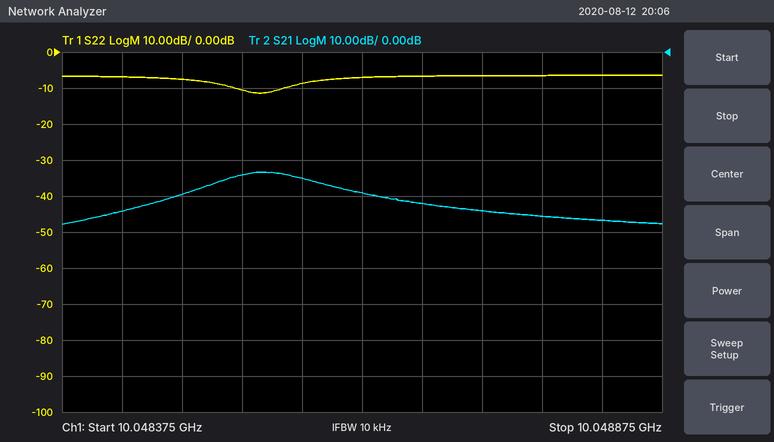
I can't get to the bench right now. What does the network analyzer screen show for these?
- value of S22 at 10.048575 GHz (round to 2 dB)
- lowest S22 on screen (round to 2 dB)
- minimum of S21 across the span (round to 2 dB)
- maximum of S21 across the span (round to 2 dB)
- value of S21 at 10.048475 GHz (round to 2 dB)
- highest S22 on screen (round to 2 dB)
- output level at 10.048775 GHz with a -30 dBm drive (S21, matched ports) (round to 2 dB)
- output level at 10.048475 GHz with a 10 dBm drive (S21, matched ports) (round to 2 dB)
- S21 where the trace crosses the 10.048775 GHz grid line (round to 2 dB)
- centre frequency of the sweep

-8 dB
-12 dB
-48 dB
-34 dB
-40 dB
-6 dB
-76 dBm
-30 dBm
-46 dB
10.048625 GHz
